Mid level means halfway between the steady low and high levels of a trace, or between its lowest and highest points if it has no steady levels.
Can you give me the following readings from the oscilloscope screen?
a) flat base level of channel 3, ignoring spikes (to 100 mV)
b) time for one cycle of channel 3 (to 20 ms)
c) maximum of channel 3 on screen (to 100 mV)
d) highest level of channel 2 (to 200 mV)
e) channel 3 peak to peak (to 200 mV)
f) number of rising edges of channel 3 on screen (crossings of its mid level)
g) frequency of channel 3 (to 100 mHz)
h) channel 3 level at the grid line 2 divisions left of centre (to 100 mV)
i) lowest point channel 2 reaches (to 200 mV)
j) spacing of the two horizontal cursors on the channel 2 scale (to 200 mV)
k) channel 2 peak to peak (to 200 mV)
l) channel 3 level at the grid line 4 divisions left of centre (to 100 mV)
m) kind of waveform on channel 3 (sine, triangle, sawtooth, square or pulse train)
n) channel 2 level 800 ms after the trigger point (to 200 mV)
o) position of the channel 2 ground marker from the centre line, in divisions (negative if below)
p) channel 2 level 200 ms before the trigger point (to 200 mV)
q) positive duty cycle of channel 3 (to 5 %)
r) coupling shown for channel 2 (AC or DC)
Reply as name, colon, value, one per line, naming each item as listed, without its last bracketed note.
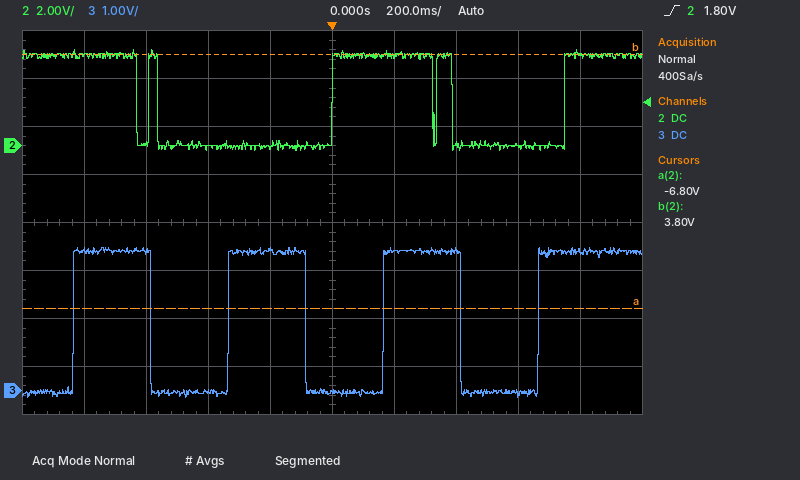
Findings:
flat base level of channel 3, ignoring spikes: 0.0 V
time for one cycle of channel 3: 500 ms
maximum of channel 3 on screen: 3.0 V
highest level of channel 2: 4.0 V
channel 3 peak to peak: 3.2 V
number of rising edges of channel 3 on screen: 4
frequency of channel 3: 2.0 Hz
channel 3 level at the grid line 2 divisions left of centre: 0.0 V
lowest point channel 2 reaches: -200 mV
spacing of the two horizontal cursors on the channel 2 scale: 10.6 V
channel 2 peak to peak: 4.2 V
channel 3 level at the grid line 4 divisions left of centre: 2.9 V
kind of waveform on channel 3: square
channel 2 level 800 ms after the trigger point: 3.8 V
position of the channel 2 ground marker from the centre line, in divisions: +1.6 div
channel 2 level 200 ms before the trigger point: 0.0 V
positive duty cycle of channel 3: 50 %
coupling shown for channel 2: DC
